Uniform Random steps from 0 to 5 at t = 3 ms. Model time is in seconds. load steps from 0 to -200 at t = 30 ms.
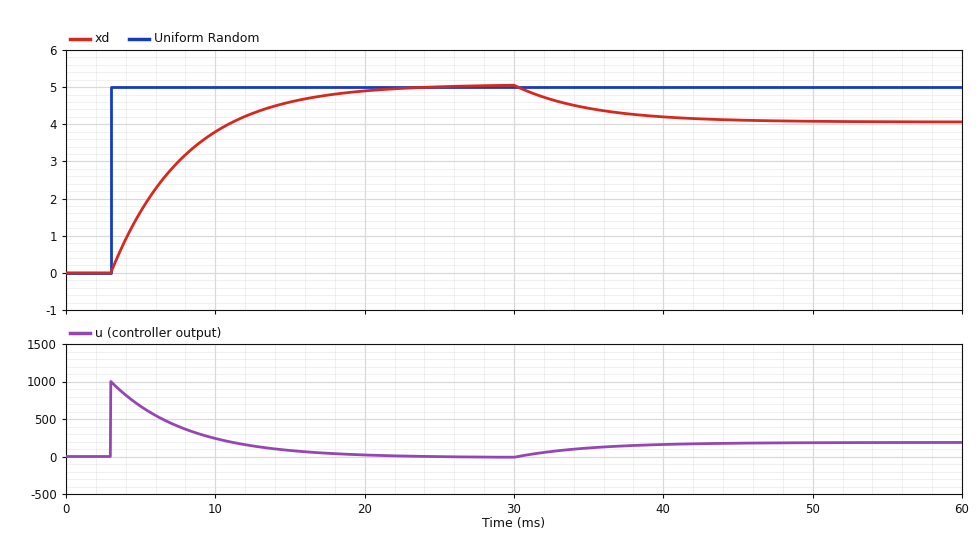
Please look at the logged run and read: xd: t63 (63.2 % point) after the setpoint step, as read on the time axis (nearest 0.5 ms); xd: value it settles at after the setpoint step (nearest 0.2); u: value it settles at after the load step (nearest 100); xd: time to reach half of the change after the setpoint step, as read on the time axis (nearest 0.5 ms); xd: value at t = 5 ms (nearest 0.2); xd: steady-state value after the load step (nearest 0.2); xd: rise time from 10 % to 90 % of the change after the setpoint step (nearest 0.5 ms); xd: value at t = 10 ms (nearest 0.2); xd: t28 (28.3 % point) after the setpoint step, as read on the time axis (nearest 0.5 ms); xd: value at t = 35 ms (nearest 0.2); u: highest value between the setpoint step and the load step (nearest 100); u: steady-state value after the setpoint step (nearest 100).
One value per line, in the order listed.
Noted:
8.0 ms
5.0
200
6.5 ms
1.6
4.0
11.0 ms
3.8
4.5 ms
4.4
1000
0
